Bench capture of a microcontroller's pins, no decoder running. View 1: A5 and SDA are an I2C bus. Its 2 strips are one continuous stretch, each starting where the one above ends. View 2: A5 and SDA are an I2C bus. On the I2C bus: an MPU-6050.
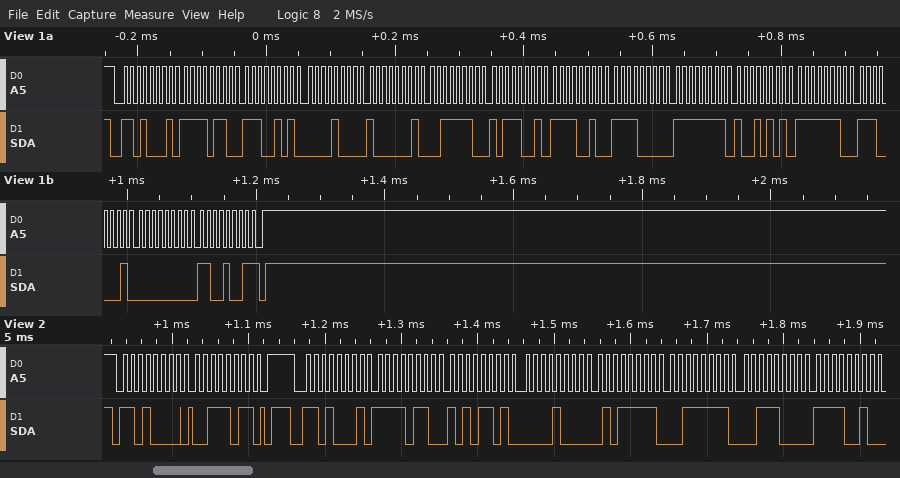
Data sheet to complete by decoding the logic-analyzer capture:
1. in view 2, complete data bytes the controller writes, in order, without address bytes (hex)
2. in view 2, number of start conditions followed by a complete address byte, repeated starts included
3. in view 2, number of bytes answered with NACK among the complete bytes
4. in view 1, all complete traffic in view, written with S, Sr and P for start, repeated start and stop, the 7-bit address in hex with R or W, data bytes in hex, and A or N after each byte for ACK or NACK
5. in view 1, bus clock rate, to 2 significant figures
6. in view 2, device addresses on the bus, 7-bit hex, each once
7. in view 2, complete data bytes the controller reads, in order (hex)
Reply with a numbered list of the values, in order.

1. 3B
2. 2
3. 0
4. S 68R A F6 A E5 A 08 A 81 A 3E A B9 A F2 A F0 A FF A 95 A FE A E1 A 00 A C9 N P
5. 100 kHz
6. 0x68
7. F6 AD 08 5F 3F 38 F2
